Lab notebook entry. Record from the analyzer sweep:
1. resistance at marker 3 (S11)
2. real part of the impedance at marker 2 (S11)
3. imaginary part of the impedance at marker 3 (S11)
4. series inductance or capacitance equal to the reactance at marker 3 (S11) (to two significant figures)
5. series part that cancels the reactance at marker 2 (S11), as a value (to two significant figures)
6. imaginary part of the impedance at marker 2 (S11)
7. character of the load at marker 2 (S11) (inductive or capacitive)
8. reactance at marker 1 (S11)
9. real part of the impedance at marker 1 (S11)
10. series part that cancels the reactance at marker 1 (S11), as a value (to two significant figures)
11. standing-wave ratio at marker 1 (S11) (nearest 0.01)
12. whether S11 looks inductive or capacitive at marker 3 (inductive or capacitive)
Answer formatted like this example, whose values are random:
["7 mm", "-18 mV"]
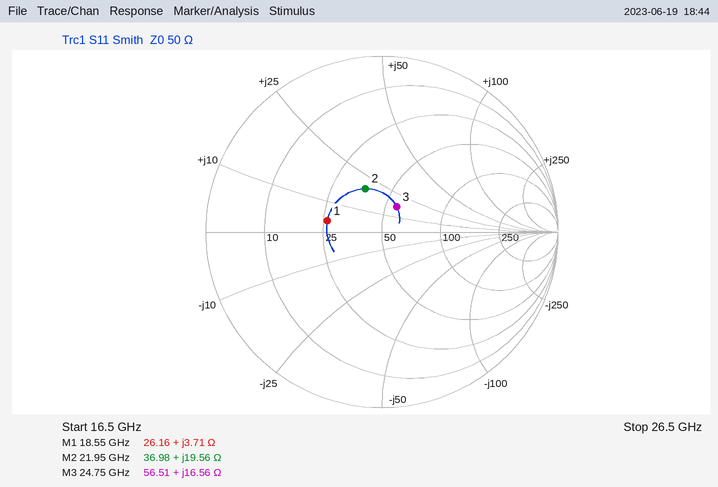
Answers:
["56.51 Ω", "36.98 Ω", "+16.56 Ω", "110 pH", "370 fF", "+19.56 Ω", "inductive", "+3.71 Ω", "26.16 Ω", "2.3 pF", "1.93", "inductive"]
